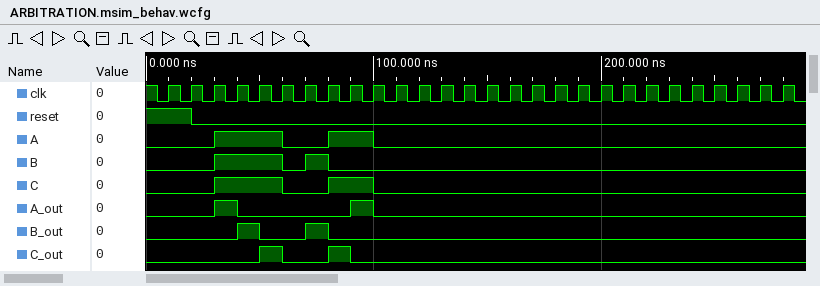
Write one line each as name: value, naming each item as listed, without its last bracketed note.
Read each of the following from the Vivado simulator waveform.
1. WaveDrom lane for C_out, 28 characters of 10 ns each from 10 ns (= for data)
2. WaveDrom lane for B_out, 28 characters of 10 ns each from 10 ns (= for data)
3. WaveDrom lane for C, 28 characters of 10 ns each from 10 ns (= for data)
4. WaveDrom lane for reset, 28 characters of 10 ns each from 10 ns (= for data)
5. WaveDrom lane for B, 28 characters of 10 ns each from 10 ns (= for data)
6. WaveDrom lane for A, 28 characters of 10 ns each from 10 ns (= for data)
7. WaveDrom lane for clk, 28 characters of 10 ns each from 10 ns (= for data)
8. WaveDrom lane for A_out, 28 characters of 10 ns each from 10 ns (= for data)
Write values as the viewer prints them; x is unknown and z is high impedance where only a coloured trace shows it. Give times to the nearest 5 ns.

WaveDrom lane for C_out, 28 characters of 10 ns each from 10 ns: {name: 'C_out', wave: '0...10.10...................'}
WaveDrom lane for B_out, 28 characters of 10 ns each from 10 ns: {name: 'B_out', wave: '0..10.10....................'}
WaveDrom lane for C, 28 characters of 10 ns each from 10 ns: {name: 'C', wave: '0.1..0.1.0..................'}
WaveDrom lane for reset, 28 characters of 10 ns each from 10 ns: {name: 'reset', wave: '10..........................'}
WaveDrom lane for B, 28 characters of 10 ns each from 10 ns: {name: 'B', wave: '0.1..010....................'}
WaveDrom lane for A, 28 characters of 10 ns each from 10 ns: {name: 'A', wave: '0.1..0.1.0..................'}
WaveDrom lane for clk, 28 characters of 10 ns each from 10 ns: {name: 'clk', wave: 'p...........................'}
WaveDrom lane for A_out, 28 characters of 10 ns each from 10 ns: {name: 'A_out', wave: '0.10....10..................'}
